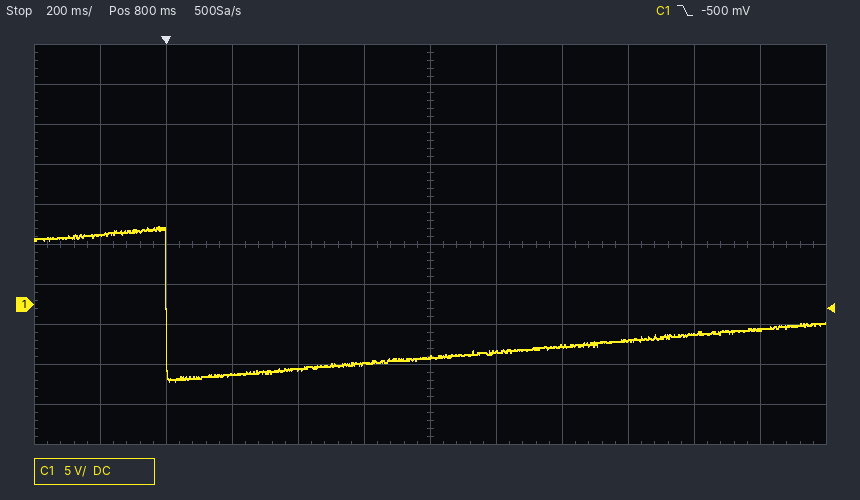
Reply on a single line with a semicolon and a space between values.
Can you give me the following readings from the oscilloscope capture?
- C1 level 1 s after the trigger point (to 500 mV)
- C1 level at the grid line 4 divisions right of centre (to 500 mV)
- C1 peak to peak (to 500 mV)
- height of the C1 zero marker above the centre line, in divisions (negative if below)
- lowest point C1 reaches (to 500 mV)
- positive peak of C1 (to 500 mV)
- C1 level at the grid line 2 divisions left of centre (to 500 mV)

-6.0 V; -3.5 V; 19.5 V; -1.5 div; -9.5 V; 10.0 V; -8.0 V
